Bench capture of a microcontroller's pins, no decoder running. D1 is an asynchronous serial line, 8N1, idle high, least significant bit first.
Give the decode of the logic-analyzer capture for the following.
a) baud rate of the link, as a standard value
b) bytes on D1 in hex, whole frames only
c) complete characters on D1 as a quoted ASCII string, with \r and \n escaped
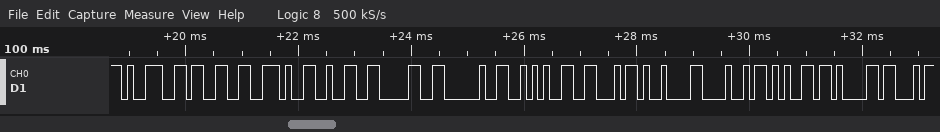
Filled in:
9600 baud
0x39 0x33 0x2E 0x32 0x30 0x20 0x2A 0x46 0x09 0x48 0x65 0x61
"93.20 *F\tHea"
